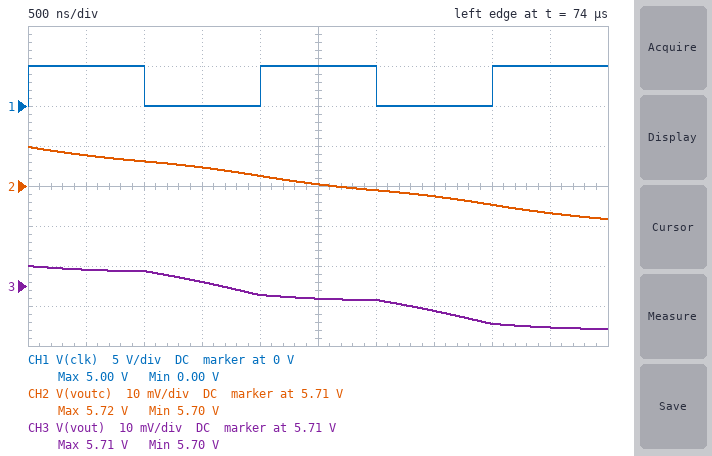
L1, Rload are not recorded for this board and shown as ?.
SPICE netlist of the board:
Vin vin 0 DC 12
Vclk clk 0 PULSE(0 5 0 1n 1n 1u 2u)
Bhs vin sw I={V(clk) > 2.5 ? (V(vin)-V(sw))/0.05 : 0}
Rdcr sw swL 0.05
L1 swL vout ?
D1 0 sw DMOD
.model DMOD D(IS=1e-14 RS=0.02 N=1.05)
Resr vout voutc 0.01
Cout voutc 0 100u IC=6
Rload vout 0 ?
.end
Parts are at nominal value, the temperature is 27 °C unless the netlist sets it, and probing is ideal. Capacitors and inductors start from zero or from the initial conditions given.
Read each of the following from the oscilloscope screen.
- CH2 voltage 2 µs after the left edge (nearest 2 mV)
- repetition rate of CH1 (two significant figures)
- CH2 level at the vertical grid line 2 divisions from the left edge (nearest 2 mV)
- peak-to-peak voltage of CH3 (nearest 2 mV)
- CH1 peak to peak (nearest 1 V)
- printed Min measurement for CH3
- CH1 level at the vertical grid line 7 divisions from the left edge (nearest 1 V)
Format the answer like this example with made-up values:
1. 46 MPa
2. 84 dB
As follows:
1. 5.712 V
2. 500 kHz
3. 5.716 V
4. 16 mV
5. 5 V
6. 5.70 V
7. 0 V
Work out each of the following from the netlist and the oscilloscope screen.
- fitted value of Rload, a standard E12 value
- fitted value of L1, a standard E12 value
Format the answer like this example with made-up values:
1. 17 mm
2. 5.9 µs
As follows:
1. 12 Ω
2. 27 µH
